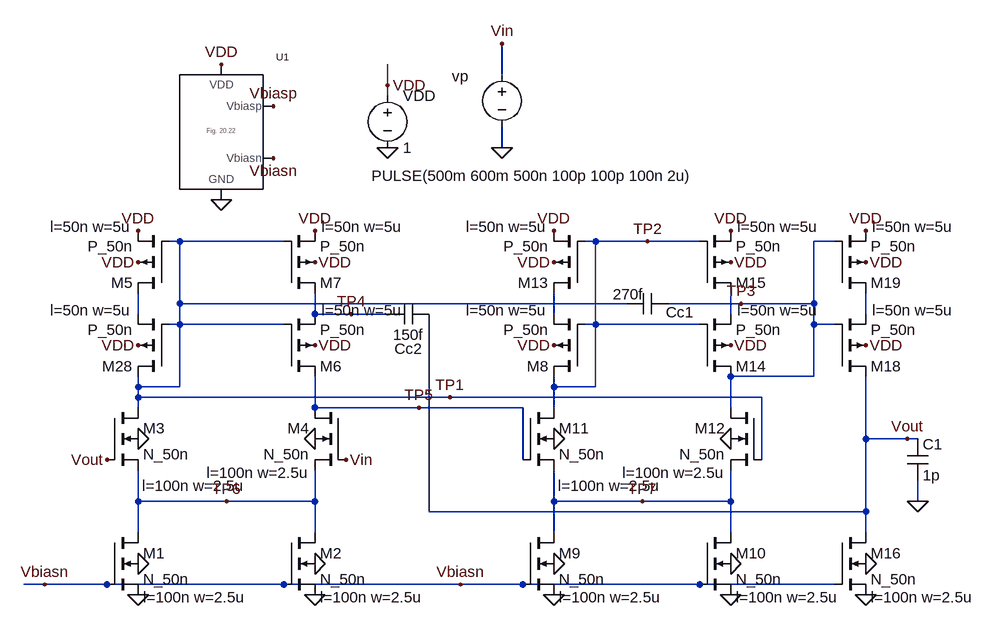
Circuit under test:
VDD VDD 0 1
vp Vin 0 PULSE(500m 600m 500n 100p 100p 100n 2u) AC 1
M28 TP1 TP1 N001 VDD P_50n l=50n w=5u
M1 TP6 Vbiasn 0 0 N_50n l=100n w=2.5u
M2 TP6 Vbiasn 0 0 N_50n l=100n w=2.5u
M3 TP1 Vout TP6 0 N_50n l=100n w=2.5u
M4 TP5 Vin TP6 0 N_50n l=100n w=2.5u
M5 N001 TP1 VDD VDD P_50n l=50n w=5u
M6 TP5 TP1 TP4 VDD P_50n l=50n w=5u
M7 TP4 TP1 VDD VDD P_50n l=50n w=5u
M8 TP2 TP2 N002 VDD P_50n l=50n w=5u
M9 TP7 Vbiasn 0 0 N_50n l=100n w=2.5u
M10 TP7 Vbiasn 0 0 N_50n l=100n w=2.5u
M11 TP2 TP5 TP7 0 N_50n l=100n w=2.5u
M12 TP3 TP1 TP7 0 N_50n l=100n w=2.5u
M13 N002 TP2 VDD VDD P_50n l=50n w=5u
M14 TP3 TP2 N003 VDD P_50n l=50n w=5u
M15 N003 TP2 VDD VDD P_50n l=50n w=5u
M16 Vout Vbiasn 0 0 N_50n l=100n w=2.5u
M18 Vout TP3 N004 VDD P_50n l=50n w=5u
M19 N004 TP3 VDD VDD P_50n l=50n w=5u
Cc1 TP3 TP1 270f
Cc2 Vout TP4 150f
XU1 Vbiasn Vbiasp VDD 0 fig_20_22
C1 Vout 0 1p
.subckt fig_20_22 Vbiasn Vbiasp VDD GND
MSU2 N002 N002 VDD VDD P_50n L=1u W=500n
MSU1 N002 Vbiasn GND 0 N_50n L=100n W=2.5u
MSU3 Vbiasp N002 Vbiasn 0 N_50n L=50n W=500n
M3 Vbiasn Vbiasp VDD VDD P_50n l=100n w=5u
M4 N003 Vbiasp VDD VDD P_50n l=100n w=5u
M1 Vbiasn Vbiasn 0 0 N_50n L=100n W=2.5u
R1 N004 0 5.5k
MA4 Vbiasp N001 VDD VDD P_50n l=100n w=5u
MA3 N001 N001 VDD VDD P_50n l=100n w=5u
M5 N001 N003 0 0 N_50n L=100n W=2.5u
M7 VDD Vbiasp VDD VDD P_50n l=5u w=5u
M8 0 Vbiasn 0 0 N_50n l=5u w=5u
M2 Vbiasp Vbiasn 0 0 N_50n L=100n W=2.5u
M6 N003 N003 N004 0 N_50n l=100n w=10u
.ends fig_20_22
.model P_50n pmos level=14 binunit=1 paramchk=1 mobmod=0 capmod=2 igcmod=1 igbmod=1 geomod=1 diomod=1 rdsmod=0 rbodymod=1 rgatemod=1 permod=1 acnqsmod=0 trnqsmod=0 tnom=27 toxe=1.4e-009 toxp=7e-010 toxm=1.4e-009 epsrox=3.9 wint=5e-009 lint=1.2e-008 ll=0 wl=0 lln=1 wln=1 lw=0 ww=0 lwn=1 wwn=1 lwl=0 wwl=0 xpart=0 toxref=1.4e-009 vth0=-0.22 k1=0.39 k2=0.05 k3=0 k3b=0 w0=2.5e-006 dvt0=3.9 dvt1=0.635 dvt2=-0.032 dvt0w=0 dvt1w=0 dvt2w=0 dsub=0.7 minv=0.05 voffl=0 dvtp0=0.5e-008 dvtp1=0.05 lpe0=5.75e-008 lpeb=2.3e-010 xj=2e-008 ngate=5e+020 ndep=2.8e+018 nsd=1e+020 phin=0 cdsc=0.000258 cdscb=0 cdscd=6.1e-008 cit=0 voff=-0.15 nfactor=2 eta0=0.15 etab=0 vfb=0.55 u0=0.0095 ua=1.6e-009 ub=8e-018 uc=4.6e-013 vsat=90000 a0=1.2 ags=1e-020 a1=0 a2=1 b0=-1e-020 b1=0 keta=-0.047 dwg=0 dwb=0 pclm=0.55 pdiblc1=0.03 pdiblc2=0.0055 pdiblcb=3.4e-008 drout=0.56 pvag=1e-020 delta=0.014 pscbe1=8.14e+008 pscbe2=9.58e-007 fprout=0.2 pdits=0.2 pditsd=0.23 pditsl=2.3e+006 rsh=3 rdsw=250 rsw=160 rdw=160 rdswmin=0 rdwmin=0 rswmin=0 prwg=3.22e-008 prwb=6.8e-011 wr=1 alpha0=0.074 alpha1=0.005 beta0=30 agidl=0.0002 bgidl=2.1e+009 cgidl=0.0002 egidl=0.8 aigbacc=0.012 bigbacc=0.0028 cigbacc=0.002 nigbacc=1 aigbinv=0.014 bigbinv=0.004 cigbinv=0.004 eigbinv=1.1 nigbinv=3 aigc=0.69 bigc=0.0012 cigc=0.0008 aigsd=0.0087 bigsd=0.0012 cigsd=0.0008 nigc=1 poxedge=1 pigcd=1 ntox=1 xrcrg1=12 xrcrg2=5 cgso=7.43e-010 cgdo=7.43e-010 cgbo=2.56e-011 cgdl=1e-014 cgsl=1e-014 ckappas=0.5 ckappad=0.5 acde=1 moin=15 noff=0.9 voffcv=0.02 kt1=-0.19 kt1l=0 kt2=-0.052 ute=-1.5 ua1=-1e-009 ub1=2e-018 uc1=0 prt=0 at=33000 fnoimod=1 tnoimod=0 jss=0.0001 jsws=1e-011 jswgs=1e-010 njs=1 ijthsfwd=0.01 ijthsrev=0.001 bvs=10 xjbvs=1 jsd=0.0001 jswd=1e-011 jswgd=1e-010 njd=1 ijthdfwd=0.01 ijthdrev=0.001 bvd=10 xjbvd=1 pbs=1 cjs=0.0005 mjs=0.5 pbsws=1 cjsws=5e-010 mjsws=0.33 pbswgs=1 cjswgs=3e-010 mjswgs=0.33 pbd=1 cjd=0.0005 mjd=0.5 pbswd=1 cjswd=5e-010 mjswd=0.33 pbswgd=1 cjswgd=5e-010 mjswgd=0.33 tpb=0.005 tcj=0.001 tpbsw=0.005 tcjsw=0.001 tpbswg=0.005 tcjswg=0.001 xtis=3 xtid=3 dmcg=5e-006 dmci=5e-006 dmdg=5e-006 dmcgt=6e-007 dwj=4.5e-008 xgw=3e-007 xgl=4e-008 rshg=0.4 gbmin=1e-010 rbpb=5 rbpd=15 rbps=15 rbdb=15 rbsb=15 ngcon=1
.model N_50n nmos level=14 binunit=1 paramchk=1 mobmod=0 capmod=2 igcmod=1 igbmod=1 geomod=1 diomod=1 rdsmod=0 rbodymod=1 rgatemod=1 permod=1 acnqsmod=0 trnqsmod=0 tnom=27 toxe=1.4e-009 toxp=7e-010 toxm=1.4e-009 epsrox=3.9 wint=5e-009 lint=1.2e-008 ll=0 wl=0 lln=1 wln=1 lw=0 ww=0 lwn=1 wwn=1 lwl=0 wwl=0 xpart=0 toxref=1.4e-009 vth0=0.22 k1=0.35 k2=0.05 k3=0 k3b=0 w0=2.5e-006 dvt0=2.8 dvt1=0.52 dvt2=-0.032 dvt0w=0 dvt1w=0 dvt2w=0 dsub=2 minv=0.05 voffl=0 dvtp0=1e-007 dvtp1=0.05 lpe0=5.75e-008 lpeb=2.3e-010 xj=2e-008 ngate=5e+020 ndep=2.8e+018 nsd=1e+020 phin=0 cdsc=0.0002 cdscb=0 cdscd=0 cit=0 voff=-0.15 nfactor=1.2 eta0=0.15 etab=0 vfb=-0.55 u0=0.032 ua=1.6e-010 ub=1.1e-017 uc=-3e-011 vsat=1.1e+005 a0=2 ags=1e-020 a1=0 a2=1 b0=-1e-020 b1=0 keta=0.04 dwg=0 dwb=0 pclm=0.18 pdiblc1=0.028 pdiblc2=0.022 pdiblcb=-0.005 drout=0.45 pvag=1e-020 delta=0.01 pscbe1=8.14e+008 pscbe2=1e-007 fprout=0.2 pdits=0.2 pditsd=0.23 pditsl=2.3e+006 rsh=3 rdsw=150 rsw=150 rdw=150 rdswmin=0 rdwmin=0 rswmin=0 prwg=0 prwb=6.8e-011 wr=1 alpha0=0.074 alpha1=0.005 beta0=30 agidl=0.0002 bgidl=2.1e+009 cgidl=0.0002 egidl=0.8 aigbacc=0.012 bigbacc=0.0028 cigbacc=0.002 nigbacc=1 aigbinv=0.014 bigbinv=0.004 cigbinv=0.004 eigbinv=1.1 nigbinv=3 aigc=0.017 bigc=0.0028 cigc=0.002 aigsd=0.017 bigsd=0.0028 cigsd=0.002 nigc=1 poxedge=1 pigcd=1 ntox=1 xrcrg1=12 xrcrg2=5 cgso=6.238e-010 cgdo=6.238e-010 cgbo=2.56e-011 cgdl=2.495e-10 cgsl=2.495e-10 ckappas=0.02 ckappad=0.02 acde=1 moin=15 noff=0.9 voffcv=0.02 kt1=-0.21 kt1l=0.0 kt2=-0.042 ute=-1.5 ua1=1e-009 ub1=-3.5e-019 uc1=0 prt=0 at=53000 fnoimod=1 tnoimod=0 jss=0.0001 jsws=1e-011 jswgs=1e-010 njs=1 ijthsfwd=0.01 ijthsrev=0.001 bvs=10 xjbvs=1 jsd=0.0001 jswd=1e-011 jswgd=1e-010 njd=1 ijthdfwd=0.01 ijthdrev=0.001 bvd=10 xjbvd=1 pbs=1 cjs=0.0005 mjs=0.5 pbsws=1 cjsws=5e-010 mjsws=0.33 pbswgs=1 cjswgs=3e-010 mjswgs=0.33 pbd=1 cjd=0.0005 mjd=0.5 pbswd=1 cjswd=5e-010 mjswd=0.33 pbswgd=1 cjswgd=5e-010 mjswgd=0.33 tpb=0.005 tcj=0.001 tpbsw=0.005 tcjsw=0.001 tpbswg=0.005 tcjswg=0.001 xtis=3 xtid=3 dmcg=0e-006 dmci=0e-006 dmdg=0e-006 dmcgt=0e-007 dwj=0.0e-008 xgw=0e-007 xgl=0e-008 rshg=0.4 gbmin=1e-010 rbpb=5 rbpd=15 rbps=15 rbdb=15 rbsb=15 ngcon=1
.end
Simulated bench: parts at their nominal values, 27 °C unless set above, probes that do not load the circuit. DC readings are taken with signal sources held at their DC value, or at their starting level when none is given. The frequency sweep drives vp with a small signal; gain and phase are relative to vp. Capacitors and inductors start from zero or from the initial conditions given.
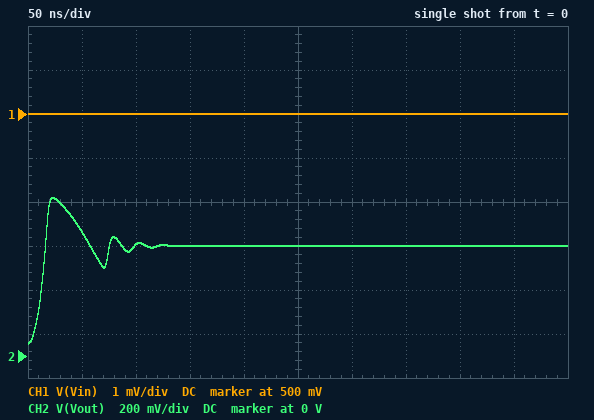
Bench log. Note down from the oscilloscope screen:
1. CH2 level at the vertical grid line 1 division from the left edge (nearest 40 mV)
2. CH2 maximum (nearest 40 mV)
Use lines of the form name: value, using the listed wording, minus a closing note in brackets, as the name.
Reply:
CH2 level at the vertical grid line 1 division from the left edge: 560 mV
CH2 maximum: 720 mV
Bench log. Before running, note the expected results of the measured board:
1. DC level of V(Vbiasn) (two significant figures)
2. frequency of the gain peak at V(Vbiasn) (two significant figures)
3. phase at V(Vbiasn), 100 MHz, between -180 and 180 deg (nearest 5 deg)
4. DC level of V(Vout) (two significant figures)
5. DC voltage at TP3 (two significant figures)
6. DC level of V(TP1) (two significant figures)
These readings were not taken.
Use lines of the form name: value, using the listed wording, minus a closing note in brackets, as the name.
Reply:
DC level of V(Vbiasn): 350 mV
frequency of the gain peak at V(Vbiasn): 46 MHz
phase at V(Vbiasn), 100 MHz, between -180 and 180 deg: -155 deg
DC level of V(Vout): 500 mV
DC voltage at TP3: 670 mV
DC level of V(TP1): 680 mV
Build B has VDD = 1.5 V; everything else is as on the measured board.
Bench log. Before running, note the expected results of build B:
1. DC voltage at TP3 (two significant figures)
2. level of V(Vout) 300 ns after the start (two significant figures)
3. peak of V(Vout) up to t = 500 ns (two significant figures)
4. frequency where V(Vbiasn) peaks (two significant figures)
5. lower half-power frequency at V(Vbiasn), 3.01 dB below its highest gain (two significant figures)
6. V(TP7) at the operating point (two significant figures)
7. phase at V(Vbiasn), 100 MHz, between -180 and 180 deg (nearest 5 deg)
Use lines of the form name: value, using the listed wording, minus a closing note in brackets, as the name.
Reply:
DC voltage at TP3: 1.2 V
level of V(Vout) 300 ns after the start: 500 mV
peak of V(Vout) up to t = 500 ns: 790 mV
frequency where V(Vbiasn) peaks: 48 MHz
lower half-power frequency at V(Vbiasn), 3.01 dB below its highest gain: 39 MHz
V(TP7) at the operating point: 660 mV
phase at V(Vbiasn), 100 MHz, between -180 and 180 deg: -150 deg
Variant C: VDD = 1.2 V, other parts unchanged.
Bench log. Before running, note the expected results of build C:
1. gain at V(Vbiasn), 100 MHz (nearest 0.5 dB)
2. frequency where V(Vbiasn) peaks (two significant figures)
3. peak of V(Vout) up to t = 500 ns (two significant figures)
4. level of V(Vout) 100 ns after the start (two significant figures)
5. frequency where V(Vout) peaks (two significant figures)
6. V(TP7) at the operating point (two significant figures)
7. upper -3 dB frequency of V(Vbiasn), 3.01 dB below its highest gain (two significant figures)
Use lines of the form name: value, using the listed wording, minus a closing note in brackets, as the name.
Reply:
gain at V(Vbiasn), 100 MHz: -47.5 dB
frequency where V(Vbiasn) peaks: 47 MHz
peak of V(Vout) up to t = 500 ns: 750 mV
level of V(Vout) 100 ns after the start: 490 mV
frequency where V(Vout) peaks: 46 MHz
V(TP7) at the operating point: 420 mV
upper -3 dB frequency of V(Vbiasn), 3.01 dB below its highest gain: 56 MHz
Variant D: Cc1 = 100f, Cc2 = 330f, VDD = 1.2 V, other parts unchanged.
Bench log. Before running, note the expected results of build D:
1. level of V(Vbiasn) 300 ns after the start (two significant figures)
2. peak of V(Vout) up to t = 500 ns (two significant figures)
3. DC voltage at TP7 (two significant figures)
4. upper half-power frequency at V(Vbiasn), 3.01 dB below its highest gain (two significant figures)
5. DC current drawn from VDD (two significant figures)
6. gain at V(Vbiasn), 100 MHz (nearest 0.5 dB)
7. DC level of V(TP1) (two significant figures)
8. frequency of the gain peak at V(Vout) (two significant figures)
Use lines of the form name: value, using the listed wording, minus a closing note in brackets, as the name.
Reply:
level of V(Vbiasn) 300 ns after the start: 350 mV
peak of V(Vout) up to t = 500 ns: 1.1 V
DC voltage at TP7: 420 mV
upper half-power frequency at V(Vbiasn), 3.01 dB below its highest gain: 110 MHz
DC current drawn from VDD: 100 µA
gain at V(Vbiasn), 100 MHz: -38.5 dB
DC level of V(TP1): 880 mV
frequency of the gain peak at V(Vout): 74 MHz
